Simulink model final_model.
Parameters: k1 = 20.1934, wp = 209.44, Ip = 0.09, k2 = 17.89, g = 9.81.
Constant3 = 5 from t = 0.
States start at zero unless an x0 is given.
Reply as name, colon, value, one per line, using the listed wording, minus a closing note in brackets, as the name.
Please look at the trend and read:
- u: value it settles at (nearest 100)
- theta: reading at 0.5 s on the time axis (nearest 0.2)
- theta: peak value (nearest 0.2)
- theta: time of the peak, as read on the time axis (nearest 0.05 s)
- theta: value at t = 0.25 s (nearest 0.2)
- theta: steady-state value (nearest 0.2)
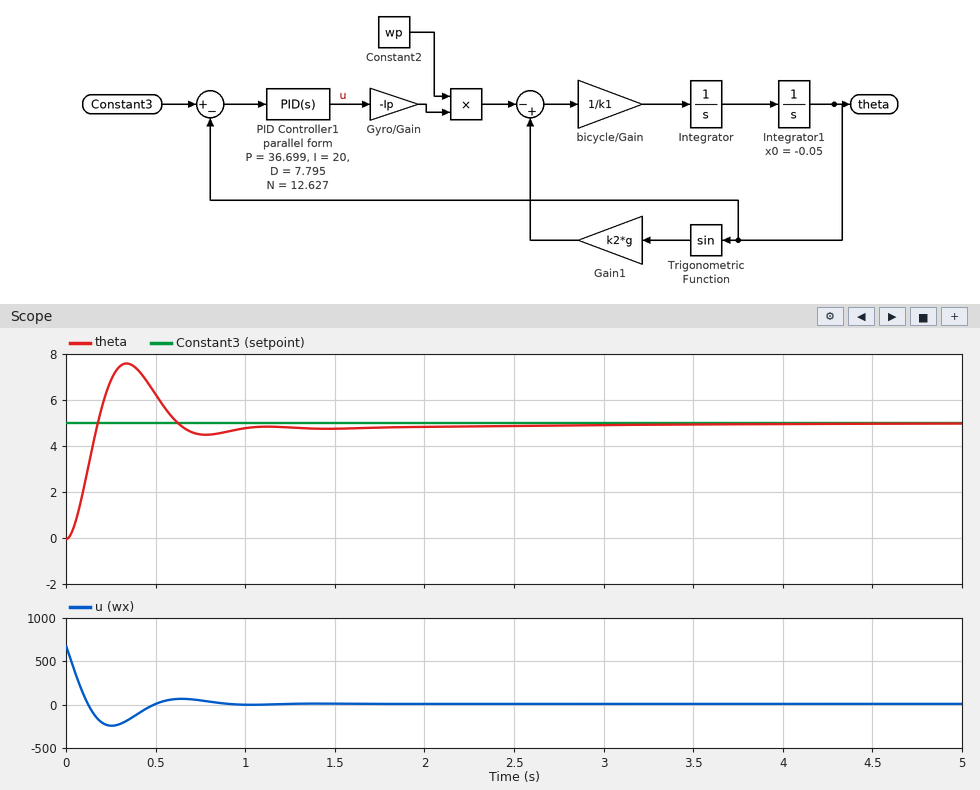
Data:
u: value it settles at: 0
theta: reading at 0.5 s on the time axis: 6.2
theta: peak value: 7.6
theta: time of the peak, as read on the time axis: 0.35 s
theta: value at t = 0.25 s: 6.8
theta: steady-state value: 5.0
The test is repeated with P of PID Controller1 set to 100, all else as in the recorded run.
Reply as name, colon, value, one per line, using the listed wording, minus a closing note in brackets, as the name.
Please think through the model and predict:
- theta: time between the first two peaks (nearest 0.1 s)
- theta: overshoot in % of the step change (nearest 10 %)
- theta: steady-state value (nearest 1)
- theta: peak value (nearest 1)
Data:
theta: time between the first two peaks: 0.5 s
theta: overshoot in % of the step change: 70 %
theta: steady-state value: 5
theta: peak value: 9
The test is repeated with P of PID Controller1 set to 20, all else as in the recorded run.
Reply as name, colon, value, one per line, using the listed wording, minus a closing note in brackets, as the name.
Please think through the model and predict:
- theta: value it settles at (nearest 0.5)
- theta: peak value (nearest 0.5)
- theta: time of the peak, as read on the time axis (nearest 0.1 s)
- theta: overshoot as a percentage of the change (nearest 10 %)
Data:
theta: value it settles at: 5.0
theta: peak value: 7.0
theta: time of the peak, as read on the time axis: 0.4 s
theta: overshoot as a percentage of the change: 40 %
